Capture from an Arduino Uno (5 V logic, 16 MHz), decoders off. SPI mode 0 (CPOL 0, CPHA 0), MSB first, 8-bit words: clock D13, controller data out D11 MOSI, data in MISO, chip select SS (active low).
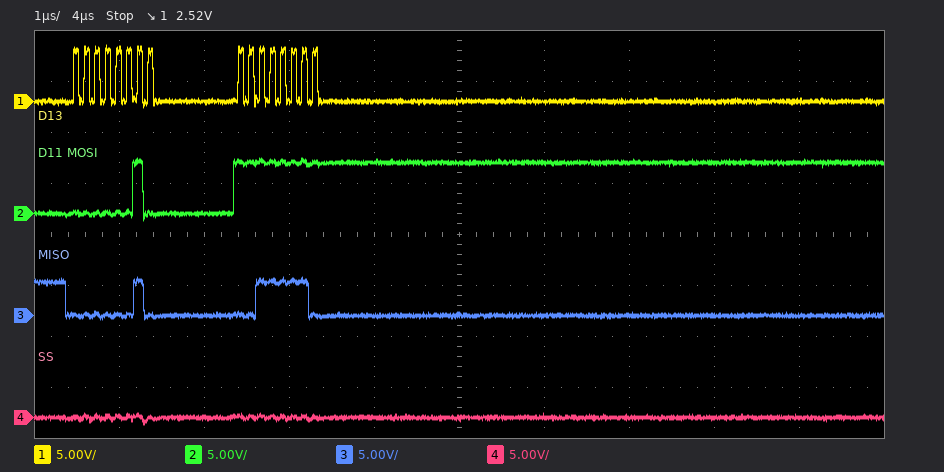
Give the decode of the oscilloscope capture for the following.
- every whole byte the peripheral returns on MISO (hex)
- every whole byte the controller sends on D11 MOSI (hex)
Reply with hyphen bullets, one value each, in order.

- 0x02 0x3E
- 0x02 0xFF
